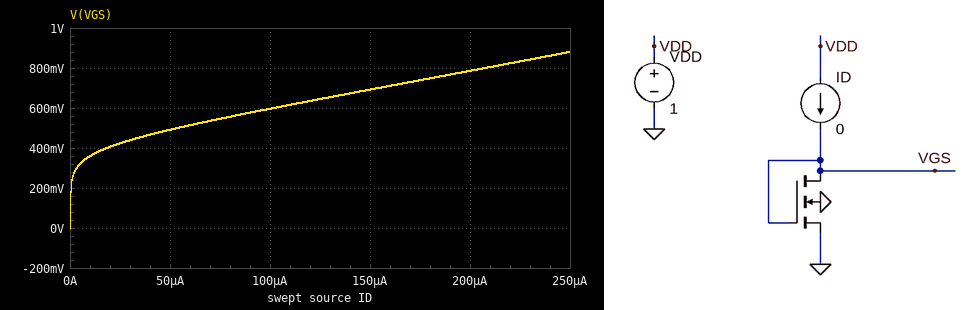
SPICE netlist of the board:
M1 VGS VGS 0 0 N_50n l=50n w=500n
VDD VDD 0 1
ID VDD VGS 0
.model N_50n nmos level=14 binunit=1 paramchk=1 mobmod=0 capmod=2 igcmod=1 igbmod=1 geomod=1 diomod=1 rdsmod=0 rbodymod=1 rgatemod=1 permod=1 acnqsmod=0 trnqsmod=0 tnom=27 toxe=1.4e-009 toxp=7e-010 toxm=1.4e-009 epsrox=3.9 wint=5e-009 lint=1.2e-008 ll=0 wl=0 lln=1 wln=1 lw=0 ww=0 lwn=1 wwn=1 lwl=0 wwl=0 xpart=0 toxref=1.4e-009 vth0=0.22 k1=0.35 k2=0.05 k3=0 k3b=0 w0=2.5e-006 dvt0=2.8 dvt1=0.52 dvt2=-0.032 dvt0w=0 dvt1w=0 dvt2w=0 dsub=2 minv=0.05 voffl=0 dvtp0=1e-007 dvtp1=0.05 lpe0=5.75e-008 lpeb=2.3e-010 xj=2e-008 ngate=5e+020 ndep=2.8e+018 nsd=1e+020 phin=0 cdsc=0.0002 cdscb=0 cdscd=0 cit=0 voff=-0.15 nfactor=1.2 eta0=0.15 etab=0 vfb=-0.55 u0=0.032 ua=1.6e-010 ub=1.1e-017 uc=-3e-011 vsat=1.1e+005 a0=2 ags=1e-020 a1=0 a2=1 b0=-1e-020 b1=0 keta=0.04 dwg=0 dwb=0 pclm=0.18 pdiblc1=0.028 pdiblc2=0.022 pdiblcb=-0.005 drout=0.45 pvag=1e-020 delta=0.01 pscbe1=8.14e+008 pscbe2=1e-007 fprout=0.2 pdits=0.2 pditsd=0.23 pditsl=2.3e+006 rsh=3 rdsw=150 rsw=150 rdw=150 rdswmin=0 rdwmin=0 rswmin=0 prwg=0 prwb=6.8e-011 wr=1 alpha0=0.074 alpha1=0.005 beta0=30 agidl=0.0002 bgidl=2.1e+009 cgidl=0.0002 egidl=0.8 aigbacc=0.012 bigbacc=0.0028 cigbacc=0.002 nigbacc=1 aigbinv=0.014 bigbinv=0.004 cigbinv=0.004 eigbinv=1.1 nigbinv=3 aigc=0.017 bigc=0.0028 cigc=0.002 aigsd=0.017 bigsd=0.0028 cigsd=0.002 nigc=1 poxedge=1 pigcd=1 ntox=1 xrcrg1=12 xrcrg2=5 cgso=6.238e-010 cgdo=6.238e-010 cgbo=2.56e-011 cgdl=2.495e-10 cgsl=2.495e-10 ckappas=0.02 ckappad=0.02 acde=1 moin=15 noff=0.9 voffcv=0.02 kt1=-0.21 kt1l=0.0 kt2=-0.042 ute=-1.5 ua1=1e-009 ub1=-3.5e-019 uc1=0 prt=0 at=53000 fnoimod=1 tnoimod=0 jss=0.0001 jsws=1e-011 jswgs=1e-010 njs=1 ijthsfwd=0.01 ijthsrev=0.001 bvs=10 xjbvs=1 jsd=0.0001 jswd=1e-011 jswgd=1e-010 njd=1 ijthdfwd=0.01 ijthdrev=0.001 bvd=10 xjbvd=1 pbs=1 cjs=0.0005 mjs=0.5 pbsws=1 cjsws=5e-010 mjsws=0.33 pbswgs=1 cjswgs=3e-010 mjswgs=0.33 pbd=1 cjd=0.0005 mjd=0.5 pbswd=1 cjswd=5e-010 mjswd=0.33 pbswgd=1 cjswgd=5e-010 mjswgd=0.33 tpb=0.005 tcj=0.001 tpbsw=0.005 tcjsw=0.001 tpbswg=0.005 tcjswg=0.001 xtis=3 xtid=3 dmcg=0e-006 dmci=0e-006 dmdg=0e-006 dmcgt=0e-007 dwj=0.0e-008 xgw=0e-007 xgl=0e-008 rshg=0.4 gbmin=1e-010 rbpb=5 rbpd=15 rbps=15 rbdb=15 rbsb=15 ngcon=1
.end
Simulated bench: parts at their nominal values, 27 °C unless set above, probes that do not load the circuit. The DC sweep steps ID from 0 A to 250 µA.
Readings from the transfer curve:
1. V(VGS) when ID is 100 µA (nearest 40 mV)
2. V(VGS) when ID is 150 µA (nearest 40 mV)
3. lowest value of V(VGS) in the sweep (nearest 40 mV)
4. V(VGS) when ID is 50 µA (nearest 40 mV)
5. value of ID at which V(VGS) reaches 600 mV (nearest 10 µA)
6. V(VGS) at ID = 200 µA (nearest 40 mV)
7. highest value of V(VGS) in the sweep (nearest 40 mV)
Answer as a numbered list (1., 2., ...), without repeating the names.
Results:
1. 600 mV
2. 680 mV
3. 0 V
4. 480 mV
5. 100 µA
6. 800 mV
7. 880 mV
